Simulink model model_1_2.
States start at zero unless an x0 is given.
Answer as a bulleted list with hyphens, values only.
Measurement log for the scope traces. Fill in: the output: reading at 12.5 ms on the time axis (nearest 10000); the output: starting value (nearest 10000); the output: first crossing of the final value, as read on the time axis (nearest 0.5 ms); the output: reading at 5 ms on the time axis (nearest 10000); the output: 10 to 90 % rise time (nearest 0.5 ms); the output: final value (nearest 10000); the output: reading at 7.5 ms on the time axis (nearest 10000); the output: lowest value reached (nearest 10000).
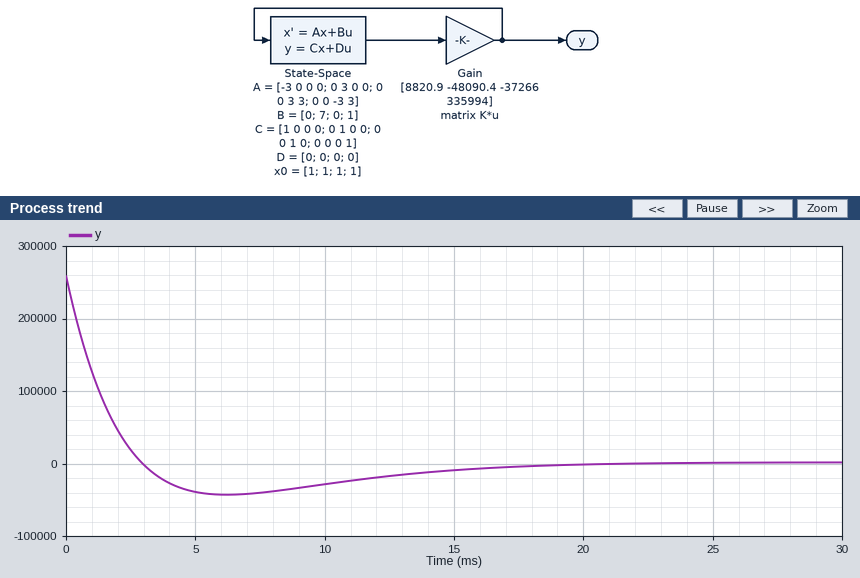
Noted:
- -20000
- 260000
- 3.0 ms
- -40000
- 2.0 ms
- 0
- -40000
- -40000
